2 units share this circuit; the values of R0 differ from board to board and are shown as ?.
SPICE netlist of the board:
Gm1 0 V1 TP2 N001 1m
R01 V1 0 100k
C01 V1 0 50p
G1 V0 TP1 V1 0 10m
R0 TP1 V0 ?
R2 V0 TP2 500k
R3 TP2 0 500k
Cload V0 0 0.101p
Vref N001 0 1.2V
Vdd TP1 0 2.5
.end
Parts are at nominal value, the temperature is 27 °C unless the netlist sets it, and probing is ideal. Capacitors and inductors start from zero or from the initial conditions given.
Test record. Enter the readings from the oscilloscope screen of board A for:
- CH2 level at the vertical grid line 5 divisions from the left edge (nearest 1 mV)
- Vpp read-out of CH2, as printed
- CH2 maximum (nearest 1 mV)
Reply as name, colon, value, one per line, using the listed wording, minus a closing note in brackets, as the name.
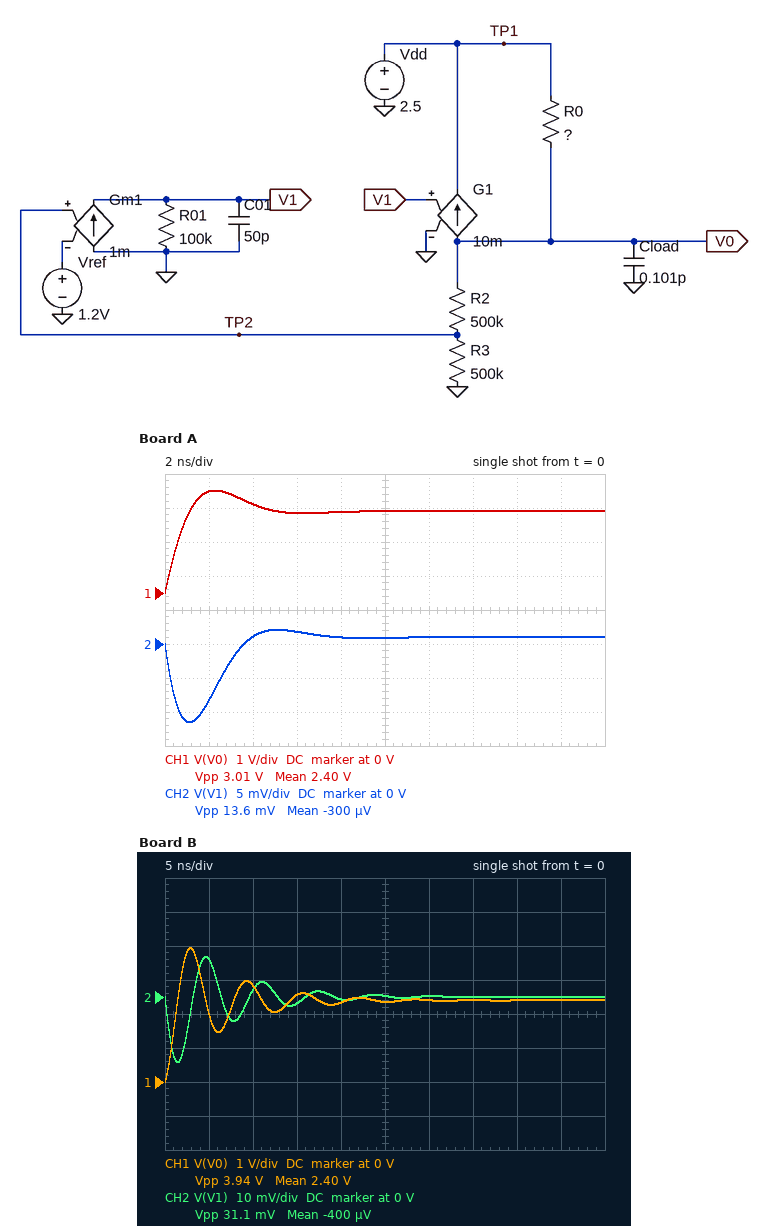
CH2 level at the vertical grid line 5 divisions from the left edge: 1 mV
Vpp read-out of CH2, as printed: 13.6 mV
CH2 maximum: 2 mV
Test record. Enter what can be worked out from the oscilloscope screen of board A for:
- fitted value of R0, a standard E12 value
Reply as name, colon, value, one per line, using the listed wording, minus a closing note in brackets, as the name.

fitted value of R0, a standard E12 value: 8.2 kΩ
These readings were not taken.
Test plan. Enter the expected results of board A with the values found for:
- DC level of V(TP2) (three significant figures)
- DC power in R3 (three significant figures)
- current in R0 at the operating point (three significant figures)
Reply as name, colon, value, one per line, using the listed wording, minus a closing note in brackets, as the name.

DC level of V(TP2): 1.20 V
DC power in R3: 2.88 µW
current in R0 at the operating point: 12.2 µA
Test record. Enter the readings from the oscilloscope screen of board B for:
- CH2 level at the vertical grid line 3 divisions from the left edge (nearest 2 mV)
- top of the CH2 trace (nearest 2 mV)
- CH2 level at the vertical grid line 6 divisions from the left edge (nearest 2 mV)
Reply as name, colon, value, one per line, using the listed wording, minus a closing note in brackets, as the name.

CH2 level at the vertical grid line 3 divisions from the left edge: -2 mV
top of the CH2 trace: 12 mV
CH2 level at the vertical grid line 6 divisions from the left edge: 0 V
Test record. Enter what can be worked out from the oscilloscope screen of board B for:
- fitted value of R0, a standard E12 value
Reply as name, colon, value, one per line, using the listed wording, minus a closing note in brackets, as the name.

fitted value of R0, a standard E12 value: 33 kΩ
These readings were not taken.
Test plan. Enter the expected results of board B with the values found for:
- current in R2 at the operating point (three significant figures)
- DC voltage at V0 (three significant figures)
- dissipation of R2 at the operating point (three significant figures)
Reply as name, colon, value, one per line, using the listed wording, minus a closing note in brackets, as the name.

current in R2 at the operating point: 2.40 µA
DC voltage at V0: 2.40 V
dissipation of R2 at the operating point: 2.88 µW
